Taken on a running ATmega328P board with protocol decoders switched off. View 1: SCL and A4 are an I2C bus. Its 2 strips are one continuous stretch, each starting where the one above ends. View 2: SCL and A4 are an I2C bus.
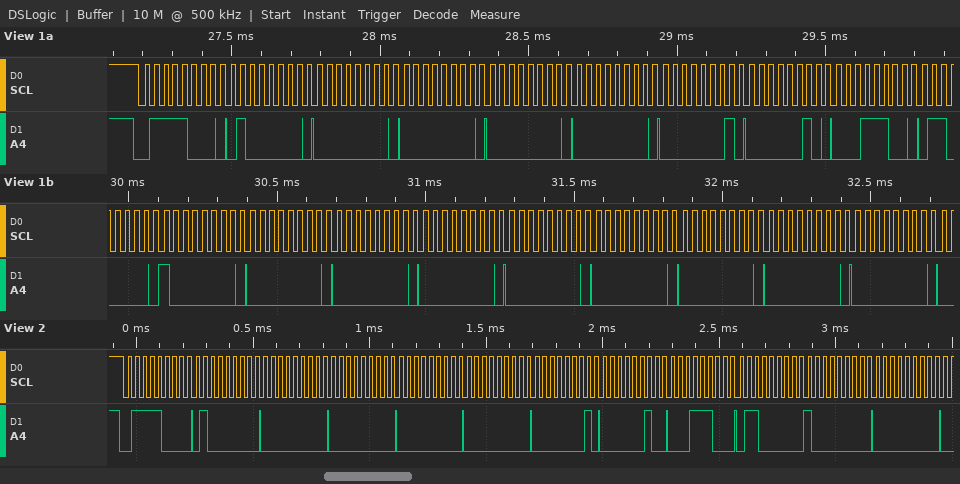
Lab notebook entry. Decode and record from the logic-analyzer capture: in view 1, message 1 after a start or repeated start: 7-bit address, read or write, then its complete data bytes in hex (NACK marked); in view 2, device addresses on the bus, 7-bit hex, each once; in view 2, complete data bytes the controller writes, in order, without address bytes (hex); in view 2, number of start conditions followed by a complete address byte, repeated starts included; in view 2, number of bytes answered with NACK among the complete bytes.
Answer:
0x3C write: 40 00 00 00 00 01 02 1C 60 80 00 00 00 00 00 00 00 00
0x3C
40 00 00 00 00 01 02 1C 60 80 00
1
0
